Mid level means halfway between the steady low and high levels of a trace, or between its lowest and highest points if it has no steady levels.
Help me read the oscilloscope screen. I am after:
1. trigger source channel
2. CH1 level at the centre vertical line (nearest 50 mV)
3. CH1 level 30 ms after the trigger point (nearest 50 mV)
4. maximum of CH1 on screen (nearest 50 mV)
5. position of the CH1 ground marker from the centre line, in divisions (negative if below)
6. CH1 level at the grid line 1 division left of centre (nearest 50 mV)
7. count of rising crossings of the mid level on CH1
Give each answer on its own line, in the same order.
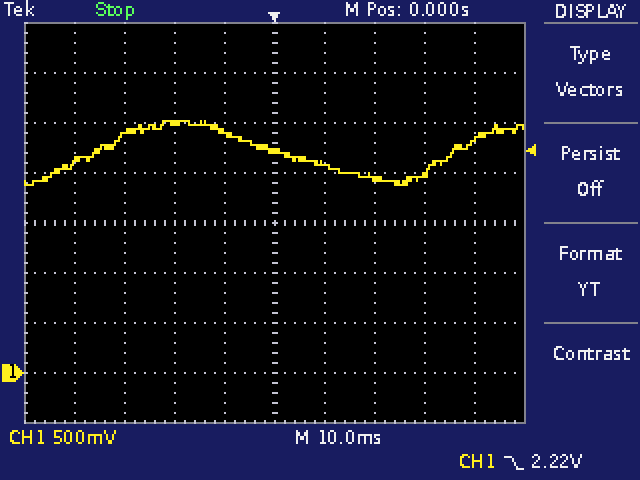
CH1
2.20 V
2.00 V
2.50 V
-3.0 div
2.40 V
2
